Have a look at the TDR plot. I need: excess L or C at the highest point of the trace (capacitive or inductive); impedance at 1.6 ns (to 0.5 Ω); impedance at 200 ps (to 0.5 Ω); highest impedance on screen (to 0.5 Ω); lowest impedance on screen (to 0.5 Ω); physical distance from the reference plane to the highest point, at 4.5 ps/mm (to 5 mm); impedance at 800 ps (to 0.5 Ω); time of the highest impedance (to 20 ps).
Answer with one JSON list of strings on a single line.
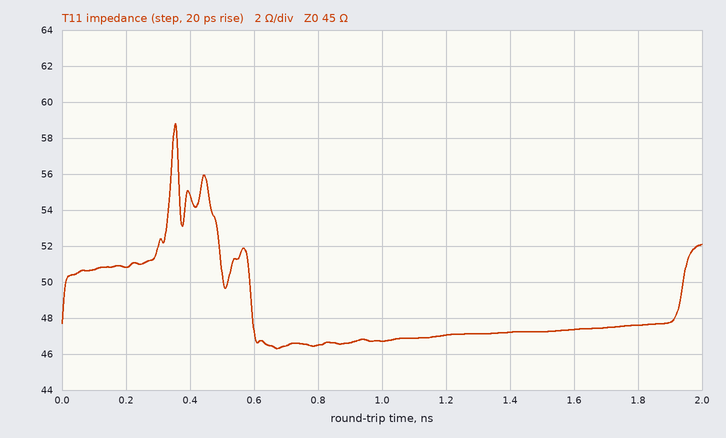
["inductive", "47.5 Ω", "51.0 Ω", "59.0 Ω", "46.5 Ω", "40 mm", "46.5 Ω", "360 ps"]
